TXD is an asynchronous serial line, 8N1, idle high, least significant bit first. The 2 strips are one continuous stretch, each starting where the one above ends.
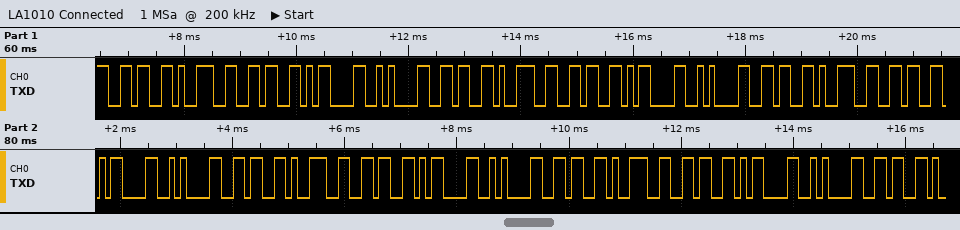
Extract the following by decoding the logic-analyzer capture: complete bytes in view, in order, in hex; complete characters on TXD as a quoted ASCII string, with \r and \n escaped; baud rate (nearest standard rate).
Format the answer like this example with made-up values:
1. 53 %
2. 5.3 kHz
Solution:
1. 36 39 36 0D 0A 36 39 36 0D 0A 36 39 36 0D 0A 36 39 36 0D 0A 36 39 36 0D 0A 36
2. "696\r\n696\r\n696\r\n696\r\n696\r\n6"
3. 9600 baud
